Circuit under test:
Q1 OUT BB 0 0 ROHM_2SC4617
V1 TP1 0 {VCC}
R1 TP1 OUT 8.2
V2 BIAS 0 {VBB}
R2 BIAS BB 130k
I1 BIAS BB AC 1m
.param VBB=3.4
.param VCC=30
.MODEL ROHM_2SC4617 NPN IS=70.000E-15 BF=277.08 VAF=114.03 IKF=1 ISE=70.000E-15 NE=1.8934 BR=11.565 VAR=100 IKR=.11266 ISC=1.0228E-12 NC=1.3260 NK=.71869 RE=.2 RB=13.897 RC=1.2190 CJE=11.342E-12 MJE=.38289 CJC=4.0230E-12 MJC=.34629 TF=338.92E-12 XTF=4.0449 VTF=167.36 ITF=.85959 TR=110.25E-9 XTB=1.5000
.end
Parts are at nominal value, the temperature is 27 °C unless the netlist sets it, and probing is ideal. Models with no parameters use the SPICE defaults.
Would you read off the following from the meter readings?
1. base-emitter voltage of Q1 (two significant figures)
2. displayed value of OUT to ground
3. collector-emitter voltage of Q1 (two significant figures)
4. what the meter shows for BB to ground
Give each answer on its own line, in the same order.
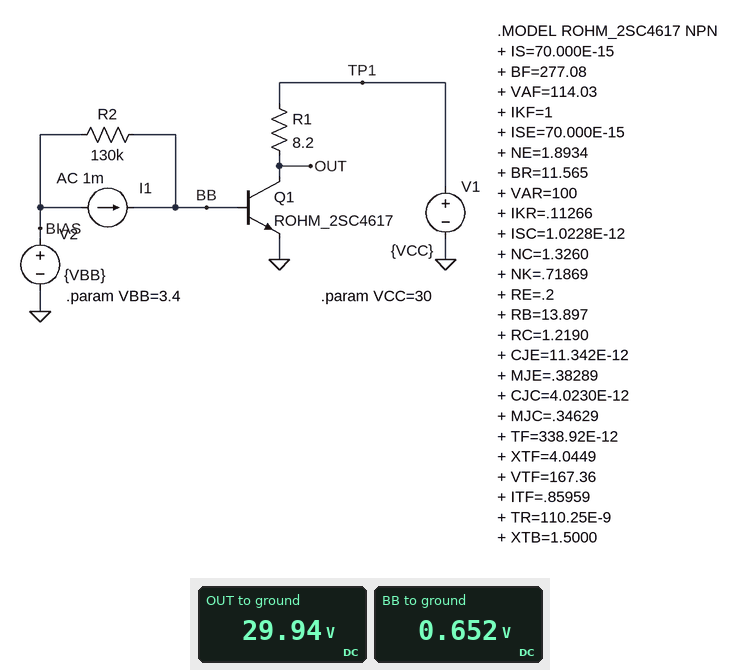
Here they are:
650 mV
29.94 V
30 V
0.652 V
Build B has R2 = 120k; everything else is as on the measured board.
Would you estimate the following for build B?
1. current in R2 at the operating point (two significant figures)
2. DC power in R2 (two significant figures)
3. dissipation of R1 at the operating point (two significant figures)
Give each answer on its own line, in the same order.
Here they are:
23 µA
63 µW
500 µW
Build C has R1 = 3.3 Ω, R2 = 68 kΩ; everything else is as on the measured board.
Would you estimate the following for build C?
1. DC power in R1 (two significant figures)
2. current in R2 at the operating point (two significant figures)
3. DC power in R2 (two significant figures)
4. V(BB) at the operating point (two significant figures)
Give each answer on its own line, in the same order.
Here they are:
620 µW
40 µA
110 µW
670 mV
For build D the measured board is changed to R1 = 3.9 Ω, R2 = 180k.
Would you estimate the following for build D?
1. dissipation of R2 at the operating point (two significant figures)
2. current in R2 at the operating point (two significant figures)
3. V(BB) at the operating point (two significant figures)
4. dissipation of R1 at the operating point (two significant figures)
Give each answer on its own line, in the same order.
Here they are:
42 µW
15 µA
640 mV
110 µW
